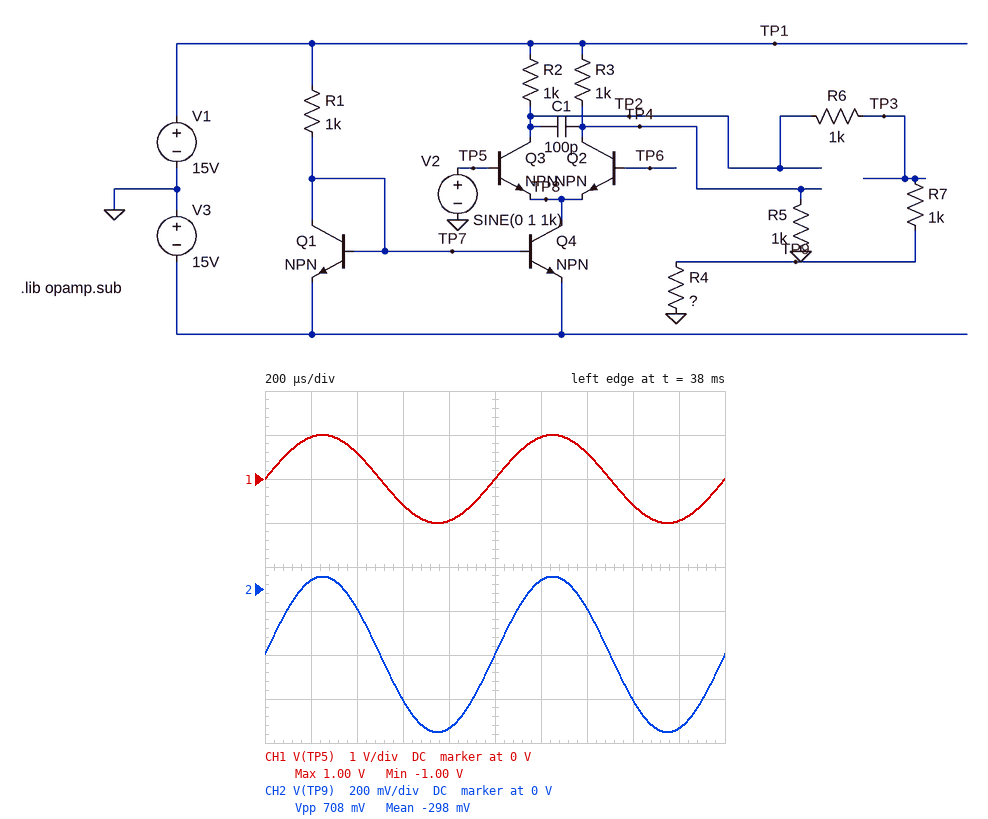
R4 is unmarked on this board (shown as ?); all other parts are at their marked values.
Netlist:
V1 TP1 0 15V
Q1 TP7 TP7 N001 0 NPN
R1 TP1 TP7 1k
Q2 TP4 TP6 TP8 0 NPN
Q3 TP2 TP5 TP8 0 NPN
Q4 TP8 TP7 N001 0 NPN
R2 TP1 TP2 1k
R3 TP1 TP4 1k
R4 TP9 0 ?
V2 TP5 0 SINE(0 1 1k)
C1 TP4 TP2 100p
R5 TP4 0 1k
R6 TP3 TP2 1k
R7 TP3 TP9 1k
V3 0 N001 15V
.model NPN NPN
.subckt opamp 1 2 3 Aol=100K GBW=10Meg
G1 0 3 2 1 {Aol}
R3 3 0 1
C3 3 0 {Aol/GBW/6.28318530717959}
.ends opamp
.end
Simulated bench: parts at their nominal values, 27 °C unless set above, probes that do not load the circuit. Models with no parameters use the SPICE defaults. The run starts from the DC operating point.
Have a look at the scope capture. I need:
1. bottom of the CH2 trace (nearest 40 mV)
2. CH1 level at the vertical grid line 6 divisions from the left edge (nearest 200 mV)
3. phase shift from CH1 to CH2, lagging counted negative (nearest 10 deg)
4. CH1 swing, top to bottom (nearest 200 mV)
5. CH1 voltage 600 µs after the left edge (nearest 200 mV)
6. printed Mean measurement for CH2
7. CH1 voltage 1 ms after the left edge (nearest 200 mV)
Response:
-640 mV
1.0 V
0 deg
2.0 V
-600 mV
-298 mV
0 V
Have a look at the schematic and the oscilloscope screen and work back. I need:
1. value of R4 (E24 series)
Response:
1.1 kΩ
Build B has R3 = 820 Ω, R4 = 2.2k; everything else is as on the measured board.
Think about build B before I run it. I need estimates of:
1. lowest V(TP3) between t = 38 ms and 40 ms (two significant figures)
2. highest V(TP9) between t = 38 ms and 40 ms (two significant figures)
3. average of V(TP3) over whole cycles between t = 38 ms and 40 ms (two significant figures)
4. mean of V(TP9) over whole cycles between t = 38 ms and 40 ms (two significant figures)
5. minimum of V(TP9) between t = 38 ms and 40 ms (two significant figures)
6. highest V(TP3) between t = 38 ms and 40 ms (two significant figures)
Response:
-1.4 V
83 mV
-640 mV
-440 mV
-960 mV
120 mV
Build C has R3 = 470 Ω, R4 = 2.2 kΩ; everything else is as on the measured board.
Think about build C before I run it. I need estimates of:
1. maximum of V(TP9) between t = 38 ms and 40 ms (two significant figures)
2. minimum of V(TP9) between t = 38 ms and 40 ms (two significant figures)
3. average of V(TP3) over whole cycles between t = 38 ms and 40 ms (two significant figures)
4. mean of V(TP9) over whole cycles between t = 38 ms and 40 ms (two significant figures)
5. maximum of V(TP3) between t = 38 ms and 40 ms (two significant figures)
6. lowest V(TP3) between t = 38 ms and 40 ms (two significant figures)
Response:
83 mV
-960 mV
-640 mV
-440 mV
120 mV
-1.4 V
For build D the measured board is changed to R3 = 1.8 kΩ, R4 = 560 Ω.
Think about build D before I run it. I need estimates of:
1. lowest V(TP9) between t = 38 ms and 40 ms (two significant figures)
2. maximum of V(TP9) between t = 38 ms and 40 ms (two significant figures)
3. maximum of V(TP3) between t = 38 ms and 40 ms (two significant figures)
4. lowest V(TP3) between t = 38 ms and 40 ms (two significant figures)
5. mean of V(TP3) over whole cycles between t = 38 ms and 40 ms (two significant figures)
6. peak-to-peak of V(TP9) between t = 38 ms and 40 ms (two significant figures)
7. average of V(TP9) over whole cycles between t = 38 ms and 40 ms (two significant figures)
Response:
-400 mV
35 mV
97 mV
-1.1 V
-510 mV
440 mV
-180 mV
